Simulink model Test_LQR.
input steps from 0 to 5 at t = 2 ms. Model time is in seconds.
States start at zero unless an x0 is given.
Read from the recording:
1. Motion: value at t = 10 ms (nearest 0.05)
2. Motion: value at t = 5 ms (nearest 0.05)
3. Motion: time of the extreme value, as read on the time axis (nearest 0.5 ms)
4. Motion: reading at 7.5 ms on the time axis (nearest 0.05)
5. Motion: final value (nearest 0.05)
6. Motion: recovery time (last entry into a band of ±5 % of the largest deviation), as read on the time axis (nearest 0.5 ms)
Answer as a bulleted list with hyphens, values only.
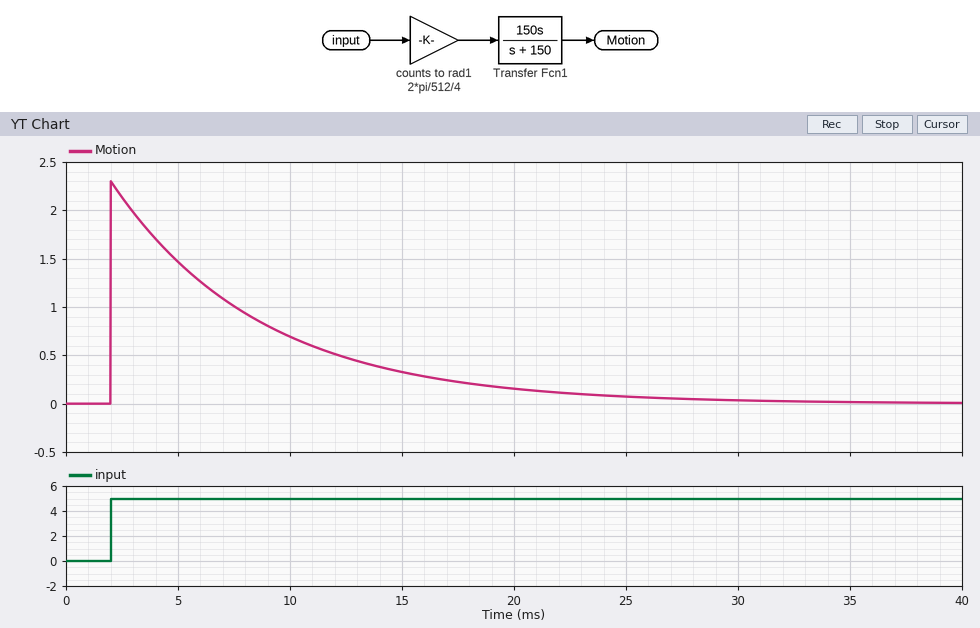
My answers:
- 0.70
- 1.45
- 2.0 ms
- 1.00
- 0.00
- 22.0 ms
